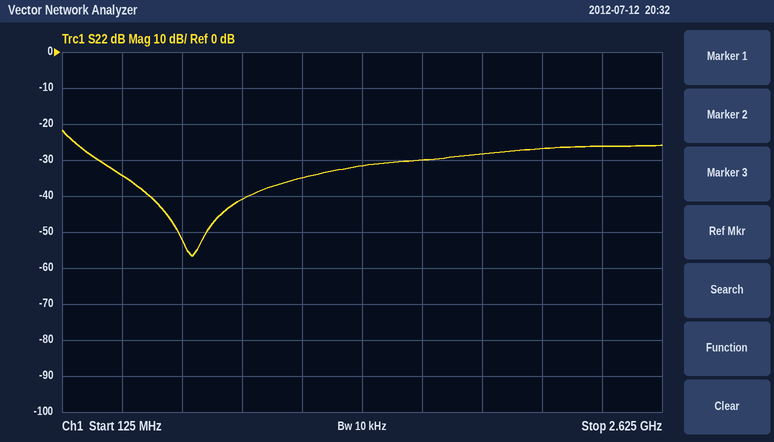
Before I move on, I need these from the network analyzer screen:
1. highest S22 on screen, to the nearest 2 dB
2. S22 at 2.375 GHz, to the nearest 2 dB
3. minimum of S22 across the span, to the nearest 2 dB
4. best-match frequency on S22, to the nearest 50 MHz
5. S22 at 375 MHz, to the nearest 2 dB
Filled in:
-22 dB
-26 dB
-56 dB
650 MHz
-34 dB
